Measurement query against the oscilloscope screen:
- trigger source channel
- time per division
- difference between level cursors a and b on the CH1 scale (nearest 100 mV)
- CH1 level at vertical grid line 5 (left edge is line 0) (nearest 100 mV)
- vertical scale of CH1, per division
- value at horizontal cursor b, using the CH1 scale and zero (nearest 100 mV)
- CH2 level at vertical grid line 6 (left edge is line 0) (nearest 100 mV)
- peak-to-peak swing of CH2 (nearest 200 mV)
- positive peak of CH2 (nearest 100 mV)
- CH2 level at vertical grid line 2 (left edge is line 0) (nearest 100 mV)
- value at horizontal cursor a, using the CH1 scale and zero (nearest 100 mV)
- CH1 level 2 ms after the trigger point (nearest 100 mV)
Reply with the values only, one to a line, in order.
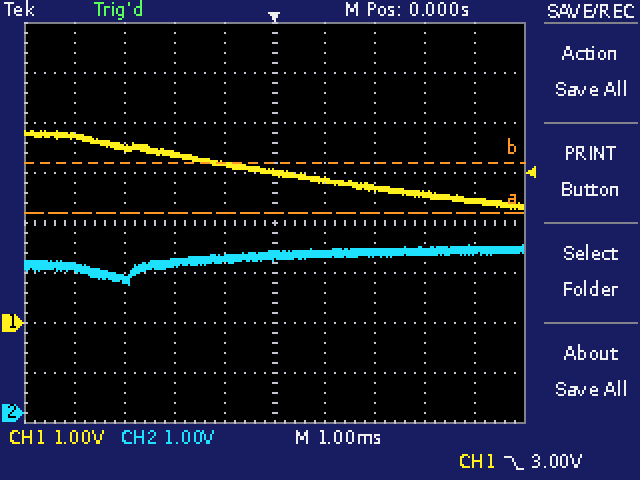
CH1
1 ms
1.0 V
3.0 V
1 V
3.2 V
3.2 V
800 mV
3.4 V
2.7 V
2.2 V
2.7 V
